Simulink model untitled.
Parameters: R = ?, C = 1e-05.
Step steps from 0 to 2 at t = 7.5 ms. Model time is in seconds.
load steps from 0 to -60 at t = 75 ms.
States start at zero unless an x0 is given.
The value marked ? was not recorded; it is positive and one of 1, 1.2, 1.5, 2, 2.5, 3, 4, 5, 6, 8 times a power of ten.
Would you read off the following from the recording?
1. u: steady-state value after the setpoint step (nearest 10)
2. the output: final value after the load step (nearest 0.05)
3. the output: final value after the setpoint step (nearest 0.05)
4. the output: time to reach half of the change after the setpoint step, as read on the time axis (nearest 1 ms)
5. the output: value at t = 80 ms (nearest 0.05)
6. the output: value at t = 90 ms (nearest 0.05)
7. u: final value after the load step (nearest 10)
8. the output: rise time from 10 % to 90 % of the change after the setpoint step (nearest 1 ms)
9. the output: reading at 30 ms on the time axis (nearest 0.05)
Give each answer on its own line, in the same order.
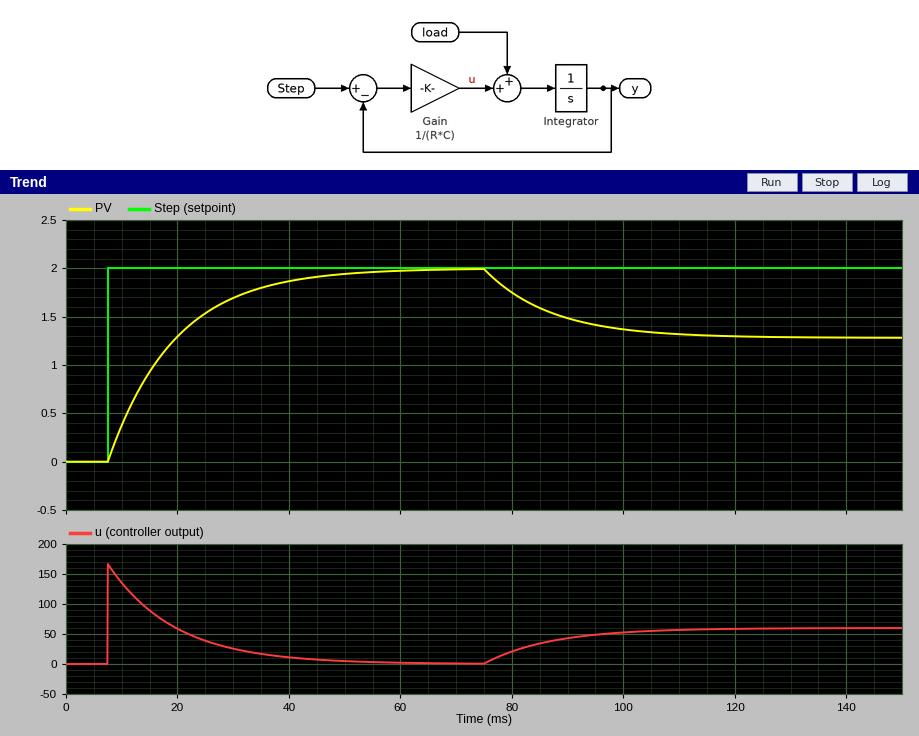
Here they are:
0
1.30
2.00
16 ms
1.75
1.50
60
26 ms
1.70
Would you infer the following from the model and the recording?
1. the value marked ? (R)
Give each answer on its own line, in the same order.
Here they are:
1200
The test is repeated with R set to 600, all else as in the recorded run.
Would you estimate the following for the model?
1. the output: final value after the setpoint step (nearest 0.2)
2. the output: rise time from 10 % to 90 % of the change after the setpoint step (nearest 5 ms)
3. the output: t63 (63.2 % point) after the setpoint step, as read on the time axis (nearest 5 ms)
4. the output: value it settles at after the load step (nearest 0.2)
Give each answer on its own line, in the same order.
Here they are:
2.0
15 ms
15 ms
1.6
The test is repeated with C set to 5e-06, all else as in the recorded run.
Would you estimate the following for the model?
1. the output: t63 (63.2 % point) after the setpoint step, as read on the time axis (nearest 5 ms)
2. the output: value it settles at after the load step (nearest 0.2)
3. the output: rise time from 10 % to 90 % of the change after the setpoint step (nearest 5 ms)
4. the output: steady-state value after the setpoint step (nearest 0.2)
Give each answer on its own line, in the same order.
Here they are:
15 ms
1.6
15 ms
2.0
